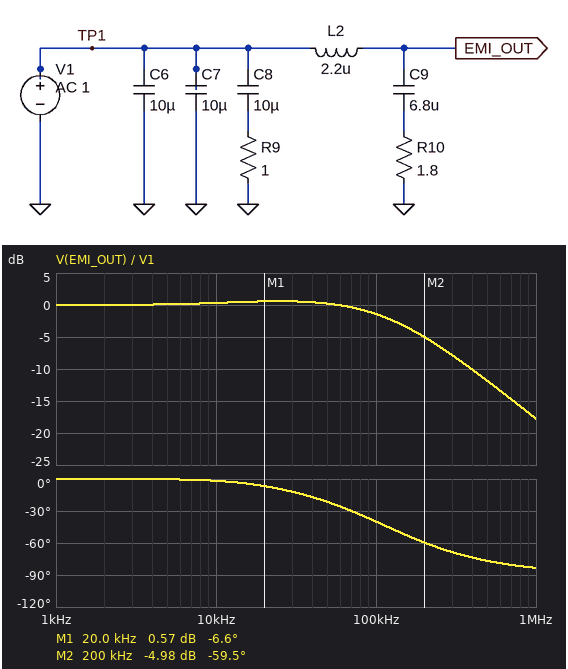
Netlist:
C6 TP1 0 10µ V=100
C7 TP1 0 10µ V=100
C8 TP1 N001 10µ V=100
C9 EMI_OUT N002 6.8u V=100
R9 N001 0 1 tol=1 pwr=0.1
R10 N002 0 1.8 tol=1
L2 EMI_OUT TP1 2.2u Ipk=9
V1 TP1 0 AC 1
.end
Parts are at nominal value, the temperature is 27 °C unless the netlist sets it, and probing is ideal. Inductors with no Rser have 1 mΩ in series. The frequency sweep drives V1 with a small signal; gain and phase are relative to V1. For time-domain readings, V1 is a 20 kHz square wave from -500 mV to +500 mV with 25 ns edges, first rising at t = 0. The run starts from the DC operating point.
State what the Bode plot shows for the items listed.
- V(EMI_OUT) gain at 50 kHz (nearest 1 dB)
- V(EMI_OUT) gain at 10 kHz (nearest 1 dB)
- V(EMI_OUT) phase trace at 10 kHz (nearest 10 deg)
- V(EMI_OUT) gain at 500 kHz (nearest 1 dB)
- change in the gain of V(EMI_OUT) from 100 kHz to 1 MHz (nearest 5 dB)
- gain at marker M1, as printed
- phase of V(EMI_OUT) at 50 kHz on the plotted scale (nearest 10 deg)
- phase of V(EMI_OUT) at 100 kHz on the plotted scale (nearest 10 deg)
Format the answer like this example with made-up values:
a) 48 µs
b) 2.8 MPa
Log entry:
a) 0 dB
b) 0 dB
c) 0 deg
d) -12 dB
e) -15 dB
f) 0.57 dB
g) -20 deg
h) -40 deg
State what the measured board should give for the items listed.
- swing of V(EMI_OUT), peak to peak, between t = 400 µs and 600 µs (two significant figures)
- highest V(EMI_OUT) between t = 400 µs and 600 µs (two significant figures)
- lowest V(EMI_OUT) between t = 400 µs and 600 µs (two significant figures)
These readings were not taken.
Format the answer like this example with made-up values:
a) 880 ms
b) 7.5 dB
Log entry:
a) 1.1 V
b) 560 mV
c) -560 mV
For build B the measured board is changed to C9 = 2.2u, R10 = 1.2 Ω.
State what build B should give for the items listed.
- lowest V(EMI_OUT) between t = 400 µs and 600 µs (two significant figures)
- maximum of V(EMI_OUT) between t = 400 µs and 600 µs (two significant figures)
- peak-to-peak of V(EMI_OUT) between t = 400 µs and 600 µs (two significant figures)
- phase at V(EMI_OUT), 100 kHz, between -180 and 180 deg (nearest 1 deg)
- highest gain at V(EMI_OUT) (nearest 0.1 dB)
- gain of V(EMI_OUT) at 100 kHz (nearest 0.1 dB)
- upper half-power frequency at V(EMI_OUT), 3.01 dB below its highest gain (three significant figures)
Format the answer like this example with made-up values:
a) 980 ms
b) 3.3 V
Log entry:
a) -750 mV
b) 750 mV
c) 1.5 V
d) -60 deg
e) 2.6 dB
f) 0.2 dB
g) 107 kHz
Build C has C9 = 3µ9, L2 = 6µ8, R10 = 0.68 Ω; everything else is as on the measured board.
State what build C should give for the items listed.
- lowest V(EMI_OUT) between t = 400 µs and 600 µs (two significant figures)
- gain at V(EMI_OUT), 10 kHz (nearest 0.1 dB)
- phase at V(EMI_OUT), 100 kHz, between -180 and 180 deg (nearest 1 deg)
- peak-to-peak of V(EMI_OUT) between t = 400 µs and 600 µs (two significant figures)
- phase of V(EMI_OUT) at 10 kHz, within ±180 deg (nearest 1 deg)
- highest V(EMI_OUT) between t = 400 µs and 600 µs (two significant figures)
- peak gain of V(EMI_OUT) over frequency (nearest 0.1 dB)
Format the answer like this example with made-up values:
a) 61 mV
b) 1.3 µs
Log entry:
a) -1.0 V
b) 0.9 dB
c) -111 deg
d) 2.0 V
e) -1 deg
f) 1.0 V
g) 7.0 dB
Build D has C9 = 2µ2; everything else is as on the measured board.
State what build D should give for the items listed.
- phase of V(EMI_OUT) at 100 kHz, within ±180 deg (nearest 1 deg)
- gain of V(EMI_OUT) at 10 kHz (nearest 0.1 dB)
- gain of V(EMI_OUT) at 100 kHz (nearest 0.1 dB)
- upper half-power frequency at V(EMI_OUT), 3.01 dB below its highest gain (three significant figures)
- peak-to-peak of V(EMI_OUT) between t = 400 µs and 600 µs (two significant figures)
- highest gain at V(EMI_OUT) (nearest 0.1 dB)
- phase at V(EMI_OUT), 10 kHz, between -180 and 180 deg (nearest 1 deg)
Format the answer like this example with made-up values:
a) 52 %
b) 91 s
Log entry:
a) -42 deg
b) 0.2 dB
c) 0.1 dB
d) 135 kHz
e) 1.3 V
f) 1.5 dB
g) 0 deg
